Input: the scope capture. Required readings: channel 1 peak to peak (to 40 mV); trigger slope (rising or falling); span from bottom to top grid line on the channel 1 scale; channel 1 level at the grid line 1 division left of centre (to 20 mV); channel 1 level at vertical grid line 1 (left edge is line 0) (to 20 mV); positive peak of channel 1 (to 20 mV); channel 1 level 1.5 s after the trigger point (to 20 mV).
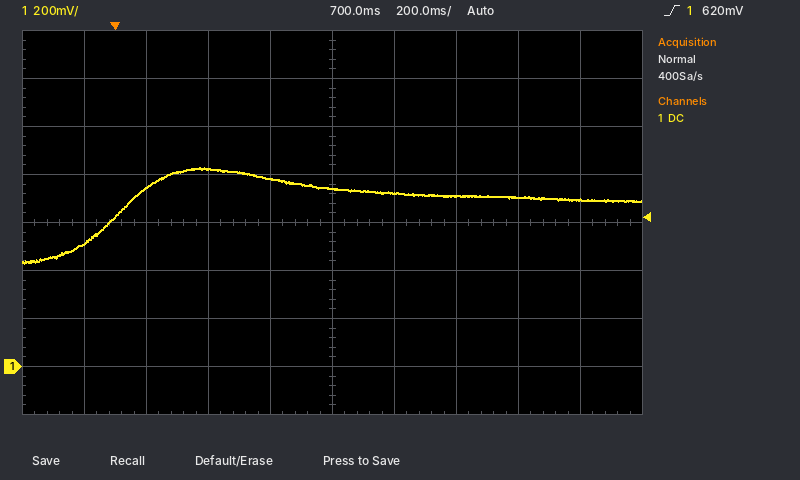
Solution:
400 mV
rising
1.6 V
780 mV
520 mV
820 mV
700 mV
